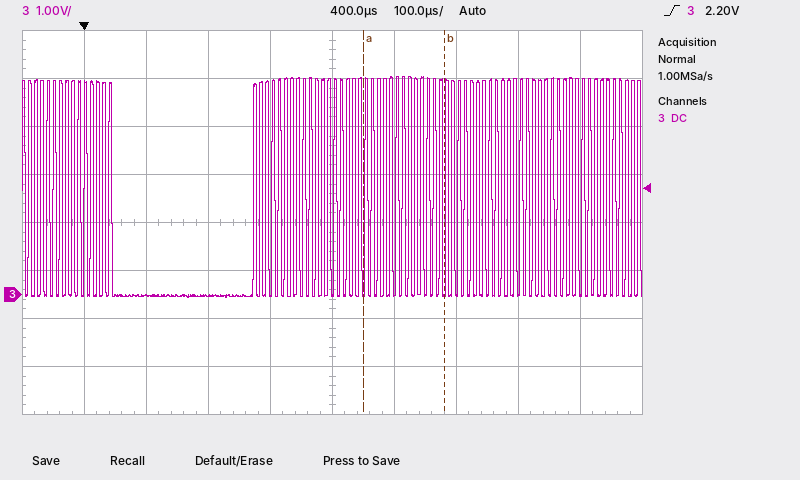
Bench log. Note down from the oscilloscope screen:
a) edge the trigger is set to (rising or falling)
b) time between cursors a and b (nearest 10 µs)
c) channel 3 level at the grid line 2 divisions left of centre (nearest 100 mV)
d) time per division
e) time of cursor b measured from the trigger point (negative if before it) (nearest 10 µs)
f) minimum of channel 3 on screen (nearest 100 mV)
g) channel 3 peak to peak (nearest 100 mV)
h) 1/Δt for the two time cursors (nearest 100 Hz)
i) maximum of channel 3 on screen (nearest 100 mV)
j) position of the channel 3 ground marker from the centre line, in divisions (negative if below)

rising
130 µs
0.0 V
100 µs
+580 µs
-100 mV
4.6 V
7.7 kHz
4.5 V
-1.5 div
